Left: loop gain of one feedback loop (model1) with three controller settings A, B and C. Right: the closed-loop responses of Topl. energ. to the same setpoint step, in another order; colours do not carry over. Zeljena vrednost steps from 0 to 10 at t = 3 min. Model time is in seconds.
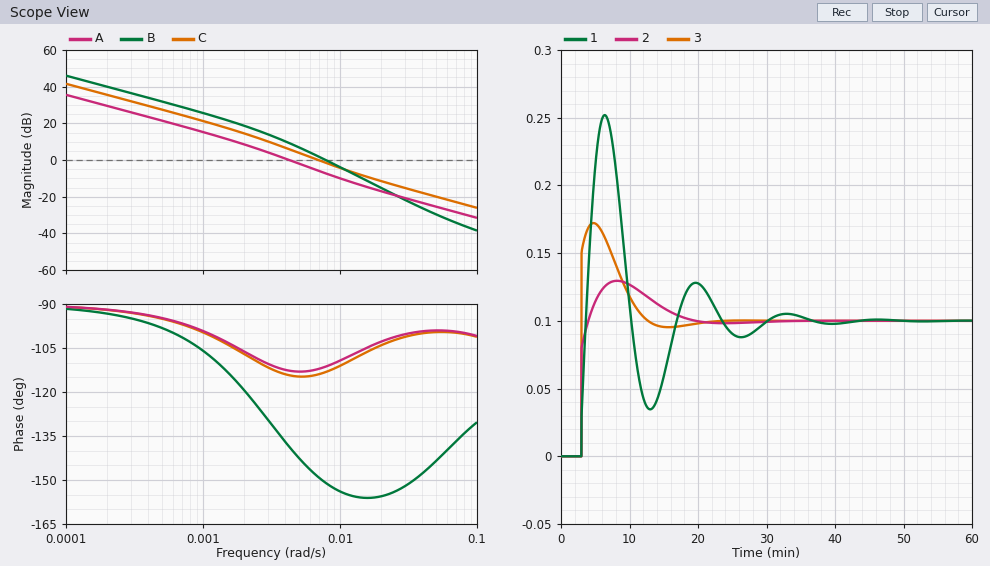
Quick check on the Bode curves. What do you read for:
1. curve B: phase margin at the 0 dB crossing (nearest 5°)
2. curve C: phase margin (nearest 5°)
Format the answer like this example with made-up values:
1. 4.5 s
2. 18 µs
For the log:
1. 30°
2. 65°
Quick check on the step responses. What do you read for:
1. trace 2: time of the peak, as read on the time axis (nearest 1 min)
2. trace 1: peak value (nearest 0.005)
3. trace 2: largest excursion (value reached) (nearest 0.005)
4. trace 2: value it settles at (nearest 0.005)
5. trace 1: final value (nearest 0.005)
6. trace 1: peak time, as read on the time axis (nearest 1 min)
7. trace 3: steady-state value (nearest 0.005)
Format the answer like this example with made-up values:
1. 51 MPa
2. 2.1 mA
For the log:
1. 8 min
2. 0.250
3. 0.130
4. 0.100
5. 0.100
6. 6 min
7. 0.100
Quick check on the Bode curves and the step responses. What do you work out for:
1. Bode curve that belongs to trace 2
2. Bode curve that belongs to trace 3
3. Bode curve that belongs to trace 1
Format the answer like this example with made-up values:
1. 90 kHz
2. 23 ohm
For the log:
1. A
2. C
3. B
